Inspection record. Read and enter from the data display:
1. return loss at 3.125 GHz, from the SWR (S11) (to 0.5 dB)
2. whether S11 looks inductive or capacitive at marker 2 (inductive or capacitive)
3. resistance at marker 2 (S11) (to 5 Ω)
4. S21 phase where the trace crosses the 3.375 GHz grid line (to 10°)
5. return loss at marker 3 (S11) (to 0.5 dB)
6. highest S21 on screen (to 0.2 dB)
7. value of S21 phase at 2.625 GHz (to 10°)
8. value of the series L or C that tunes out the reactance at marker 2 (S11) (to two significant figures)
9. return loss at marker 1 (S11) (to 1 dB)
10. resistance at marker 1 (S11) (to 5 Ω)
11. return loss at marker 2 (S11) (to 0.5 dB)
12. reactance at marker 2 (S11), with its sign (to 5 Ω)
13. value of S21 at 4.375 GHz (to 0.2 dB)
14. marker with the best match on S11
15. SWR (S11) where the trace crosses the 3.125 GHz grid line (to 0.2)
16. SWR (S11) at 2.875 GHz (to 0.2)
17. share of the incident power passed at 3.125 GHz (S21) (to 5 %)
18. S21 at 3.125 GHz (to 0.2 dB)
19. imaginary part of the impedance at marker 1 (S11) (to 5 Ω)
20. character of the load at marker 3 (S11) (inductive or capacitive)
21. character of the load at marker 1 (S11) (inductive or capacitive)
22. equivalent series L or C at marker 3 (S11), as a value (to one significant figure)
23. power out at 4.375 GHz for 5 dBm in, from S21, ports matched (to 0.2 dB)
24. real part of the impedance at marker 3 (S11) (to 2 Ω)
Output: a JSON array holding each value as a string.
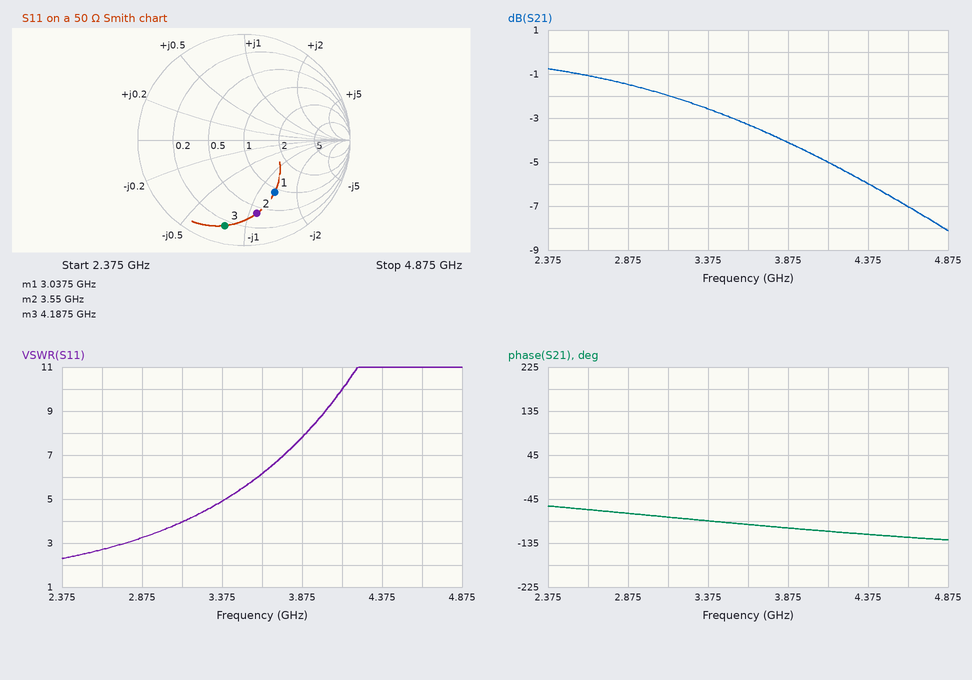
["4.5 dB", "capacitive", "20 Ω", "-90°", "1.5 dB", "-0.8 dB", "-70°", "2.5 nH", "5 dB", "45 Ω", "3.0 dB", "-55 Ω", "-6.0 dB", "marker 1", "4.0", "3.2", "65 %", "-2.0 dB", "-65 Ω", "capacitive", "capacitive", "1.0 pF", "-1.0 dBm", "8 Ω"]
